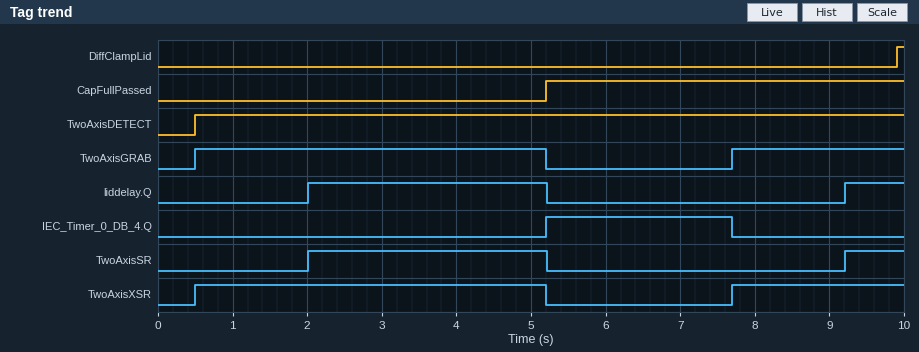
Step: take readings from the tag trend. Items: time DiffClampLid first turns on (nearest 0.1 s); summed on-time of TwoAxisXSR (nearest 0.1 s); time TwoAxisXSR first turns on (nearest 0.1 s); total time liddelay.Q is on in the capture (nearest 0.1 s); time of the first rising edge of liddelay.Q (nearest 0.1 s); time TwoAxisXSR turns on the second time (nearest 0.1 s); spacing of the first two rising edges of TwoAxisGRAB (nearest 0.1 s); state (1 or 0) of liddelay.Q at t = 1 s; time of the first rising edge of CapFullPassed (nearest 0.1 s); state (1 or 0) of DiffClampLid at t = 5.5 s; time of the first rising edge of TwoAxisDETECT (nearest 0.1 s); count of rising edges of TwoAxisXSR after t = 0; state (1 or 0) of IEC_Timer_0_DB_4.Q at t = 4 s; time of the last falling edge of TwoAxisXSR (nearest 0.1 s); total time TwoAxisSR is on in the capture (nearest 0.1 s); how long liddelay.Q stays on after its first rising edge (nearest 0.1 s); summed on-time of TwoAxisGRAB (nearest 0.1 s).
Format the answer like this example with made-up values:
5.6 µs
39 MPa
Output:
9.9 s
7.0 s
0.5 s
4.0 s
2.0 s
7.7 s
7.2 s
0
5.2 s
0
0.5 s
2
0
5.2 s
4.0 s
3.2 s
7.0 s
